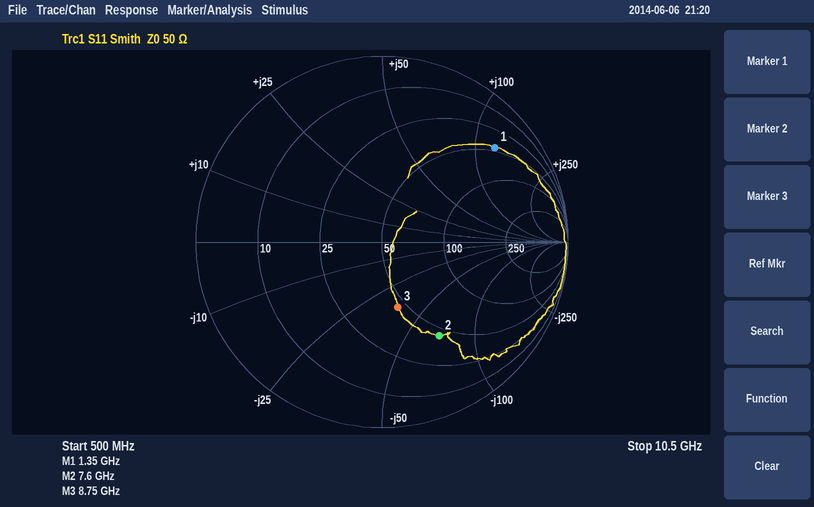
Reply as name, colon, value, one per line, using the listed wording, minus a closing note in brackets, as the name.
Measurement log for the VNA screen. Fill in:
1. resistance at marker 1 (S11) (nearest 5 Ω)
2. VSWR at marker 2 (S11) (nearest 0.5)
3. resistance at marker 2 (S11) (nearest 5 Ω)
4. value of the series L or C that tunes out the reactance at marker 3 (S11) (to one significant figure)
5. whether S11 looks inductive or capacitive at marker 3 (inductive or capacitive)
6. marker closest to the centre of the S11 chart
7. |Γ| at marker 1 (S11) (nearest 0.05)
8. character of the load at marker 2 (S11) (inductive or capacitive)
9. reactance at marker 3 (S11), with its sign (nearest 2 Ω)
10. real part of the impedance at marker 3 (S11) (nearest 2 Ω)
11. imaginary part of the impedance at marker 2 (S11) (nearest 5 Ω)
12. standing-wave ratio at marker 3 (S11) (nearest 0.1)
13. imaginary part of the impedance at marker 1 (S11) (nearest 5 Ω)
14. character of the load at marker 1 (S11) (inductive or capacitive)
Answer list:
resistance at marker 1 (S11): 45 Ω
VSWR at marker 2 (S11): 4.0
resistance at marker 2 (S11): 45 Ω
value of the series L or C that tunes out the reactance at marker 3 (S11): 700 pH
whether S11 looks inductive or capacitive at marker 3: capacitive
marker closest to the centre of the S11 chart: marker 3
|Γ| at marker 1 (S11): 0.80
character of the load at marker 2 (S11): capacitive
reactance at marker 3 (S11), with its sign: -36 Ω
real part of the impedance at marker 3 (S11): 46 Ω
imaginary part of the impedance at marker 2 (S11): -70 Ω
standing-wave ratio at marker 3 (S11): 2.1
imaginary part of the impedance at marker 1 (S11): +125 Ω
character of the load at marker 1 (S11): inductive
